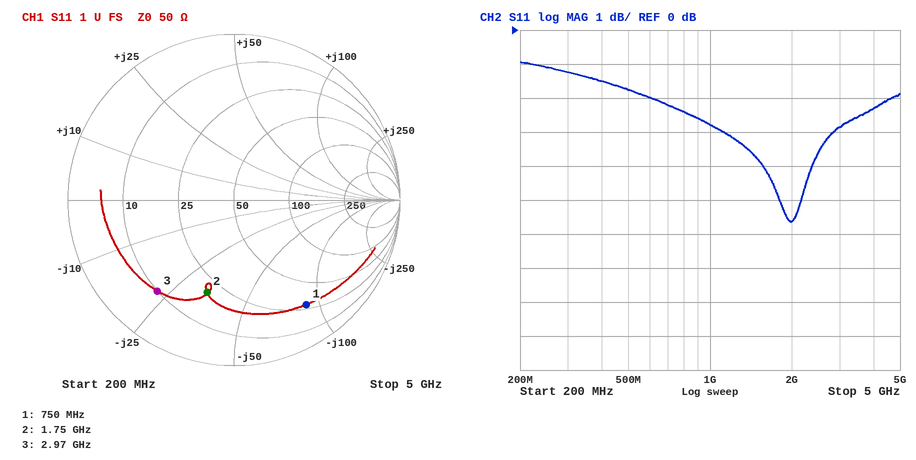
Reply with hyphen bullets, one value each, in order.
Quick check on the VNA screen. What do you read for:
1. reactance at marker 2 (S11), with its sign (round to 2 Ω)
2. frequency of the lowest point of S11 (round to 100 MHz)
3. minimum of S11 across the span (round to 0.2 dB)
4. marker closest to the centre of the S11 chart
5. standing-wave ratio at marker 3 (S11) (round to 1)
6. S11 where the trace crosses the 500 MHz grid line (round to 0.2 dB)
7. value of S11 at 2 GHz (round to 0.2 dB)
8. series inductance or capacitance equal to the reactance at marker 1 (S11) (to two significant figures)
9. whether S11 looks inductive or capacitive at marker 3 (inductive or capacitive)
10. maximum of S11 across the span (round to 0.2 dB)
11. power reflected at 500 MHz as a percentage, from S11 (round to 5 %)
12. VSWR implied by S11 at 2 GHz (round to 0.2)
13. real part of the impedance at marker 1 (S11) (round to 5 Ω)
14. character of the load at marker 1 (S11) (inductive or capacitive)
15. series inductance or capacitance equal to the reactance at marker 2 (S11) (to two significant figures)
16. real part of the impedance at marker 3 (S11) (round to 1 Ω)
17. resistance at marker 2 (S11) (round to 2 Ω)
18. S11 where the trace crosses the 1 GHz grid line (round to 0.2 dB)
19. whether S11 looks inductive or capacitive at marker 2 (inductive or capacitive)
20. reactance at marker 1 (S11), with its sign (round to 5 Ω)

- -34 Ω
- 2.0 GHz
- -5.6 dB
- marker 2
- 6
- -1.8 dB
- -5.6 dB
- 2.4 pF
- capacitive
- -1.0 dB
- 65 %
- 3.2
- 30 Ω
- capacitive
- 2.7 pF
- 10 Ω
- 20 Ω
- -2.8 dB
- capacitive
- -90 Ω
